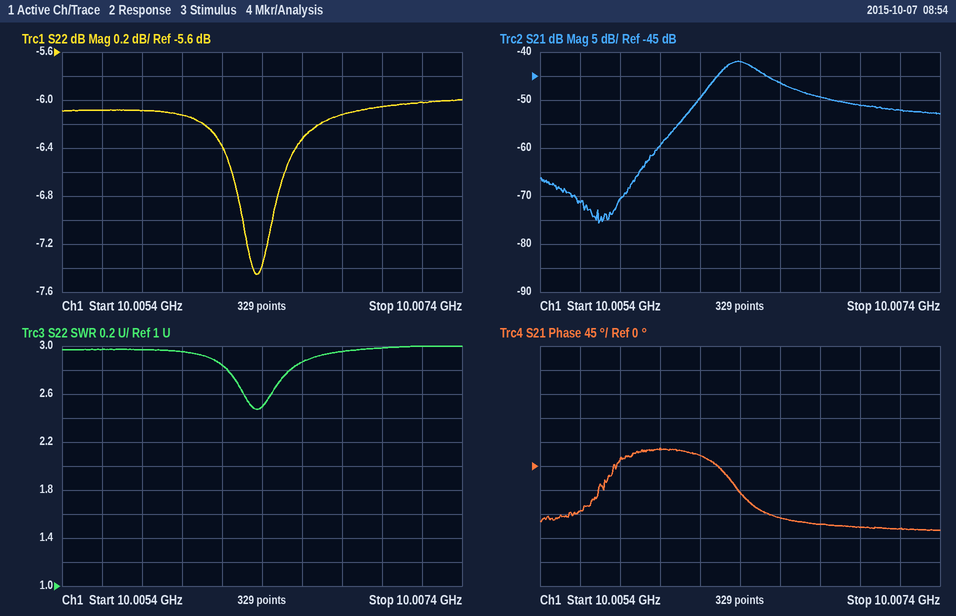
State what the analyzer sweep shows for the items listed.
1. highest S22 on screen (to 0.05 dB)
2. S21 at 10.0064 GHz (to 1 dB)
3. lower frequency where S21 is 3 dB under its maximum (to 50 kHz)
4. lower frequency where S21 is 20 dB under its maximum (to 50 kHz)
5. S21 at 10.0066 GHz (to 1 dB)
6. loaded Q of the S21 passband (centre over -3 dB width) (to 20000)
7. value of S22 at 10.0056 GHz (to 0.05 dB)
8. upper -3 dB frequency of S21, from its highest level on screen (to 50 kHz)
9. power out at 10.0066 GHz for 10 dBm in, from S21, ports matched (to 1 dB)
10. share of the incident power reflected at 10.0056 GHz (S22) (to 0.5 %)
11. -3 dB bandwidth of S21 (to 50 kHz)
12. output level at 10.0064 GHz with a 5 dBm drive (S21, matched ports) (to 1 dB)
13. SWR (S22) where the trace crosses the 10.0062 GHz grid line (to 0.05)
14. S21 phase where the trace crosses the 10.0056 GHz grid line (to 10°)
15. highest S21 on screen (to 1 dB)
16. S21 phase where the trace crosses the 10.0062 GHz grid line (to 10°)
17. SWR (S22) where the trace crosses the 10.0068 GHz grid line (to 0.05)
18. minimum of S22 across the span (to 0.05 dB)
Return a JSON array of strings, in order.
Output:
["-6.00 dB", "-42 dB", "10.00630 GHz", "10.00595 GHz", "-46 dB", "40000", "-6.10 dB", "10.00655 GHz", "-36 dBm", "24.5 %", "250 kHz", "-37 dBm", "2.85", "-80°", "-42 dB", "20°", "2.95", "-7.45 dB"]
